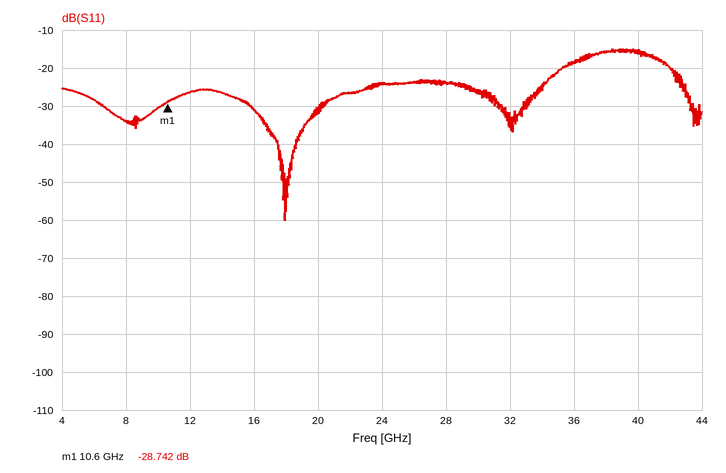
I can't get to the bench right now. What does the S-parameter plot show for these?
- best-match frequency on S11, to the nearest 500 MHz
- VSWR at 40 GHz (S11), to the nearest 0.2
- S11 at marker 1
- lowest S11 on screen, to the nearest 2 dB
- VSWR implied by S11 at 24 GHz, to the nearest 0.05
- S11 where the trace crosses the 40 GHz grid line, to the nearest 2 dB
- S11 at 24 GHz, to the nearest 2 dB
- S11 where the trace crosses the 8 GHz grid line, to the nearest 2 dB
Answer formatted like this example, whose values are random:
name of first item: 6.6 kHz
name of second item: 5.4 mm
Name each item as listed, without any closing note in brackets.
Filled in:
best-match frequency on S11, to the nearest 500 MHz: 18.0 GHz
VSWR at 40 GHz (S11), to the nearest 0.2: 1.4
S11 at marker 1: -28.742 dB
lowest S11 on screen, to the nearest 2 dB: -60 dB
VSWR implied by S11 at 24 GHz, to the nearest 0.05: 1.15
S11 where the trace crosses the 40 GHz grid line, to the nearest 2 dB: -16 dB
S11 at 24 GHz, to the nearest 2 dB: -24 dB
S11 where the trace crosses the 8 GHz grid line, to the nearest 2 dB: -34 dB
